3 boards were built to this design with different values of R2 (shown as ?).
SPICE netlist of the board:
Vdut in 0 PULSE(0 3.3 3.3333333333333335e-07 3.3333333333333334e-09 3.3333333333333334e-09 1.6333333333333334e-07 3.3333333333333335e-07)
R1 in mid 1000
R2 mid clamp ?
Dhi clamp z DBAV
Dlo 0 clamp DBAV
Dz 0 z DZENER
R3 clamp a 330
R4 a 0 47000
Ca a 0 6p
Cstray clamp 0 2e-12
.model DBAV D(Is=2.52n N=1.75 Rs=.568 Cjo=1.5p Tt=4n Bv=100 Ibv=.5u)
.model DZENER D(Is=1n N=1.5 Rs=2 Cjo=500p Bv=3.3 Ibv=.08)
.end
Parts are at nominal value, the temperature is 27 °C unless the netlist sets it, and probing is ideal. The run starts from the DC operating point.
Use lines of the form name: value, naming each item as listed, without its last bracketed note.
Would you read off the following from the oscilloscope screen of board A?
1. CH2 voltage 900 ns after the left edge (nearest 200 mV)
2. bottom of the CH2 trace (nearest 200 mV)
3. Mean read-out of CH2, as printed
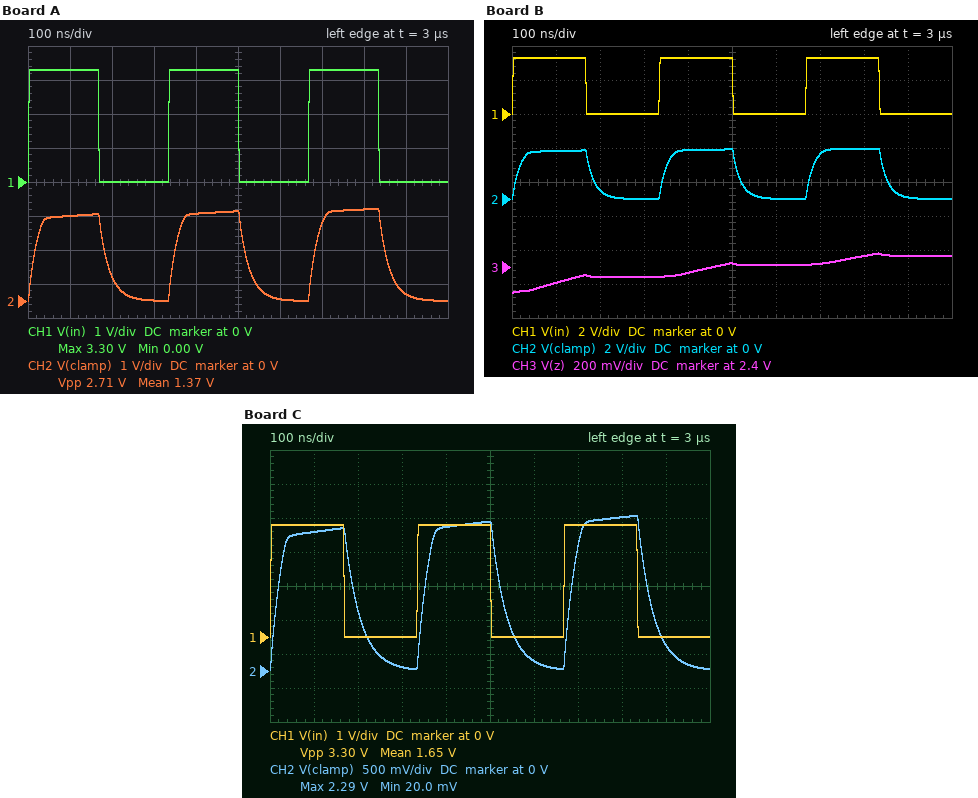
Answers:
CH2 voltage 900 ns after the left edge: 200 mV
bottom of the CH2 trace: 0 V
Mean read-out of CH2, as printed: 1.37 V
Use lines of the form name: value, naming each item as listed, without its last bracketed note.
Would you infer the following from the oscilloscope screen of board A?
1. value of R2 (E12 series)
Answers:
value of R2: 1.5 kΩ
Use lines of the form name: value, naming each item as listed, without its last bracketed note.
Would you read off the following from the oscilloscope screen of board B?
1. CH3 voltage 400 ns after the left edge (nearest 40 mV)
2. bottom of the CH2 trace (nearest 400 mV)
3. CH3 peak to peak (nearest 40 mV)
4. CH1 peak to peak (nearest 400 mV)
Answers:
CH3 voltage 400 ns after the left edge: 2.36 V
bottom of the CH2 trace: 0 V
CH3 peak to peak: 240 mV
CH1 peak to peak: 3.2 V
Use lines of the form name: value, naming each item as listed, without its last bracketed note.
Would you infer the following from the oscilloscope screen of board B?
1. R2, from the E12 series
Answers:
R2, from the E12 series: 820 Ω
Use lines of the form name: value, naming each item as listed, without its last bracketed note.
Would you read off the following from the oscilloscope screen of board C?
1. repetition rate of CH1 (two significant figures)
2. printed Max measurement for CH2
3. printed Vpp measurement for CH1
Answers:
repetition rate of CH1: 3.0 MHz
printed Max measurement for CH2: 2.29 V
printed Vpp measurement for CH1: 3.30 V
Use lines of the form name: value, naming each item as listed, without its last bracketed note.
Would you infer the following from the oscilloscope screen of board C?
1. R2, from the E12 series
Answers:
R2, from the E12 series: 2.7 kΩ
